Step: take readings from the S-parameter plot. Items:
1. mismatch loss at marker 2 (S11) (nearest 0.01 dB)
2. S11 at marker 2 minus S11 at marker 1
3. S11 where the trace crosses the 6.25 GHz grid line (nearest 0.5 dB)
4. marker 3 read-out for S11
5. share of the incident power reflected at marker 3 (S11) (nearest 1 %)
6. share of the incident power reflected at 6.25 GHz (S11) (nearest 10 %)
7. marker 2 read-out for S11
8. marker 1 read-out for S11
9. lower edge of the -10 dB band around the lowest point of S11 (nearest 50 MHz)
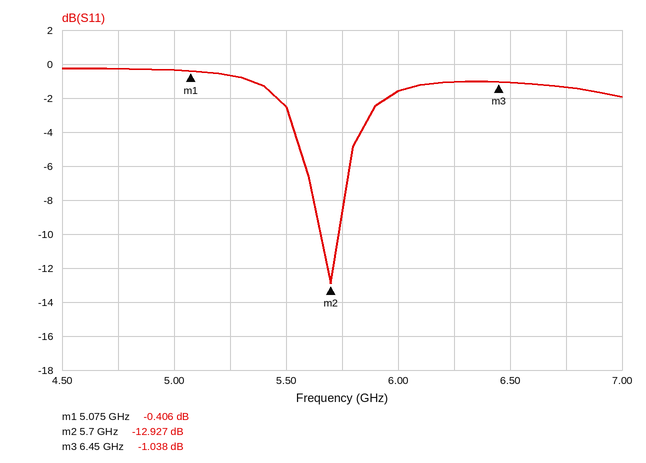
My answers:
0.23 dB
-12.521 dB
-1.0 dB
-1.038 dB
79 %
80 %
-12.927 dB
-0.406 dB
5.65 GHz
